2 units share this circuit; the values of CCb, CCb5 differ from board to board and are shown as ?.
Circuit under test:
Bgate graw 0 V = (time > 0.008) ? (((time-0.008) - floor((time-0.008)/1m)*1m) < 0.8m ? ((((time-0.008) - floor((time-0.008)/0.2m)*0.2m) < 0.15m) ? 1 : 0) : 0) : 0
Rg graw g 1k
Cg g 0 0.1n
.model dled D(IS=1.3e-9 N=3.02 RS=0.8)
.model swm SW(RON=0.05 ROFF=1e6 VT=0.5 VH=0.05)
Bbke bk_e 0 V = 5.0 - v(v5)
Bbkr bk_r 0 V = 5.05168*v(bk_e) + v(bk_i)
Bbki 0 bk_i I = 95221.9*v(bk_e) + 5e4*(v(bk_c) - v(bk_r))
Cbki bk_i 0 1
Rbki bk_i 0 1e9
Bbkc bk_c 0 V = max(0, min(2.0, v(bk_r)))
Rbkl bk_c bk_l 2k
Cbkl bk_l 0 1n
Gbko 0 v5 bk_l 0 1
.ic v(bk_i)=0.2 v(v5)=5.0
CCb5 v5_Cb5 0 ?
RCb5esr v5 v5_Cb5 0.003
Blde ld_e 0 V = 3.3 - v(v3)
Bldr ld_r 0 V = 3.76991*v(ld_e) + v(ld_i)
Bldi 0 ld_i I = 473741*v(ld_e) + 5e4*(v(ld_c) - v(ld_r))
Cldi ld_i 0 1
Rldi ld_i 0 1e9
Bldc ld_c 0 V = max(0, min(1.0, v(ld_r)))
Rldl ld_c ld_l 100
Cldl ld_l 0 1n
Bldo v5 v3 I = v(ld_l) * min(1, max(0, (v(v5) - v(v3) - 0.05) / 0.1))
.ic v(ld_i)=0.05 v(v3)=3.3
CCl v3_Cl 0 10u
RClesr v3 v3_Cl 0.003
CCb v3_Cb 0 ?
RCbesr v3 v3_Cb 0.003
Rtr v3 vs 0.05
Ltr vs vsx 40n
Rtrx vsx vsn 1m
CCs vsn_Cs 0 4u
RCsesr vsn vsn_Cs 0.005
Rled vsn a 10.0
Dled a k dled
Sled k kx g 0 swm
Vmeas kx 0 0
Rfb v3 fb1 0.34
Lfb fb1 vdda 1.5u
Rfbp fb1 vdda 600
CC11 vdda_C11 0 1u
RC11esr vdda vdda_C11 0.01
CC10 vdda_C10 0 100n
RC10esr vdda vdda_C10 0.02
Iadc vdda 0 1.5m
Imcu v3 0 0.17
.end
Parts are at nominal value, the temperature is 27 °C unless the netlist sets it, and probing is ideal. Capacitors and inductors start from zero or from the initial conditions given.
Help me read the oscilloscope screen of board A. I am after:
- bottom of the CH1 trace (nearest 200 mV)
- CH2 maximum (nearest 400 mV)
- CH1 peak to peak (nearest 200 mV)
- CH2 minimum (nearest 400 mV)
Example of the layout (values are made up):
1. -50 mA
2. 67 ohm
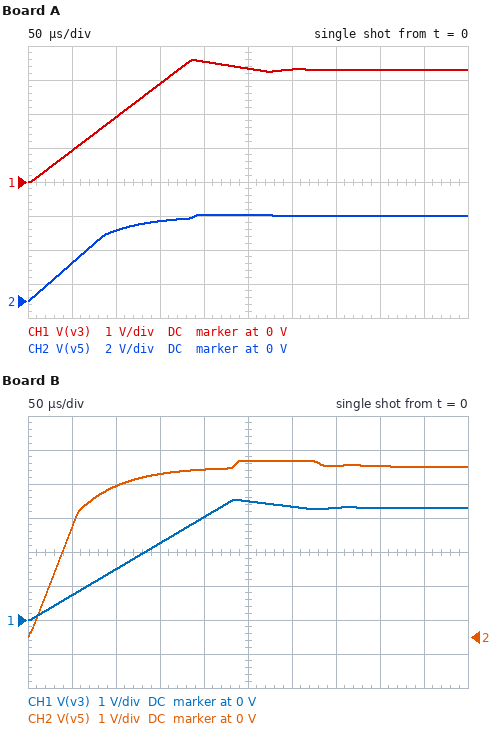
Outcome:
1. 0 V
2. 5.2 V
3. 3.6 V
4. 0 V
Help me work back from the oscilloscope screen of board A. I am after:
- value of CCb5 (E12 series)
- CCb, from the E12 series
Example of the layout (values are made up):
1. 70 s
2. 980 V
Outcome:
1. 22 µF
2. 27 µF
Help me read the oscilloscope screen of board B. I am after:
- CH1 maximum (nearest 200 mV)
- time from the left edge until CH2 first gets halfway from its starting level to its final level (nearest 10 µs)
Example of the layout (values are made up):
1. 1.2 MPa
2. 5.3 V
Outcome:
1. 3.6 V
2. 40 µs
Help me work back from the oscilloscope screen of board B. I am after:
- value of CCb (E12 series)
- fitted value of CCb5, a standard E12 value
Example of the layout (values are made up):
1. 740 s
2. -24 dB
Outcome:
1. 39 µF
2. 15 µF
